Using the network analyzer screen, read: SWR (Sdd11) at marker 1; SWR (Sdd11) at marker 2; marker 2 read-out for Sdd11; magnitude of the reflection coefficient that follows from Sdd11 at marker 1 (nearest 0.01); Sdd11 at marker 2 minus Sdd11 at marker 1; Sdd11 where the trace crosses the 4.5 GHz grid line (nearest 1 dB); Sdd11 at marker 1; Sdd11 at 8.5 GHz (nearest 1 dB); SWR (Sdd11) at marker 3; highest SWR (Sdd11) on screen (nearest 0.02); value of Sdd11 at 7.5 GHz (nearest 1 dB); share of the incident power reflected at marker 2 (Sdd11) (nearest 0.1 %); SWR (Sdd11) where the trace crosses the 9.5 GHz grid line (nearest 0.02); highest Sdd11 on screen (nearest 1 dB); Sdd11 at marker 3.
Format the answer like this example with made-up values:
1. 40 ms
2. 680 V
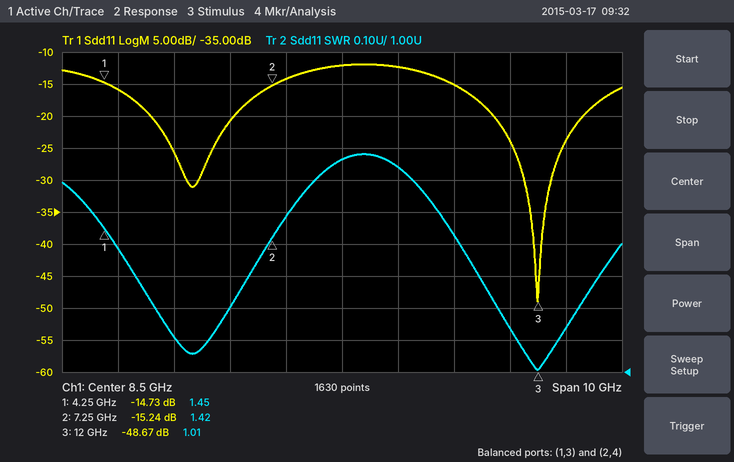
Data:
1. 1.45
2. 1.42
3. -15.24 dB
4. 0.18
5. -0.51 dB
6. -16 dB
7. -14.73 dB
8. -12 dB
9. 1.01
10. 1.68
11. -14 dB
12. 3.0 %
13. 1.64
14. -12 dB
15. -48.67 dB
